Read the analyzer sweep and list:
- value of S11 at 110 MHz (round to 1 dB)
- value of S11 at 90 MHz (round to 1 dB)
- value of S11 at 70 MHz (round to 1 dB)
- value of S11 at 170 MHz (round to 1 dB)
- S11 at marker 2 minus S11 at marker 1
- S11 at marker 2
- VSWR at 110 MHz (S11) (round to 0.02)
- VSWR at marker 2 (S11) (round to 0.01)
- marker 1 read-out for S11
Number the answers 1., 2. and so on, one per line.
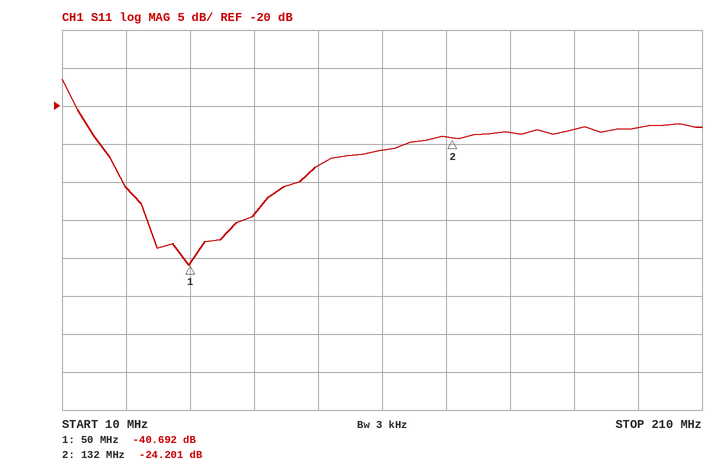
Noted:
1. -26 dB
2. -28 dB
3. -34 dB
4. -23 dB
5. 16.491 dB
6. -24.201 dB
7. 1.10
8. 1.13
9. -40.692 dB
